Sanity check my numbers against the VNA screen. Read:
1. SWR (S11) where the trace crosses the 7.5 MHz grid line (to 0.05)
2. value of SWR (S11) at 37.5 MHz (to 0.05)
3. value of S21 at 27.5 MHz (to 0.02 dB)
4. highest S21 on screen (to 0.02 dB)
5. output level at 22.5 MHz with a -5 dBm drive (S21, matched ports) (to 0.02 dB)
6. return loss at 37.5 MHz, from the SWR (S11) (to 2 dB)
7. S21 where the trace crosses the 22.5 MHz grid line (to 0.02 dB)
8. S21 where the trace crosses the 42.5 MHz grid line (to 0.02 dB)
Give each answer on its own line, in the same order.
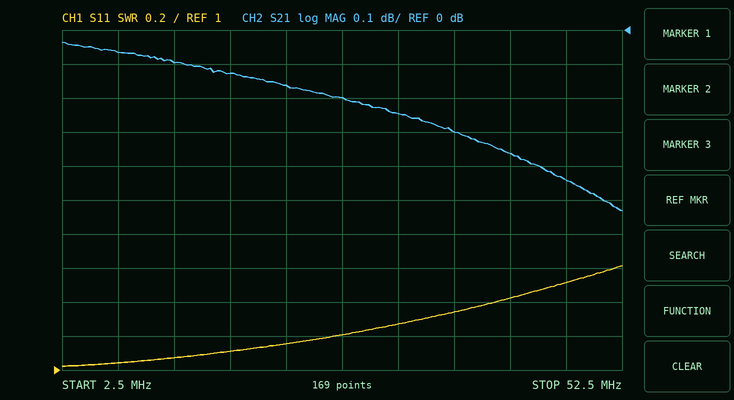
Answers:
1.05
1.35
-0.20 dB
-0.04 dB
-5.16 dBm
16 dB
-0.16 dB
-0.36 dB
